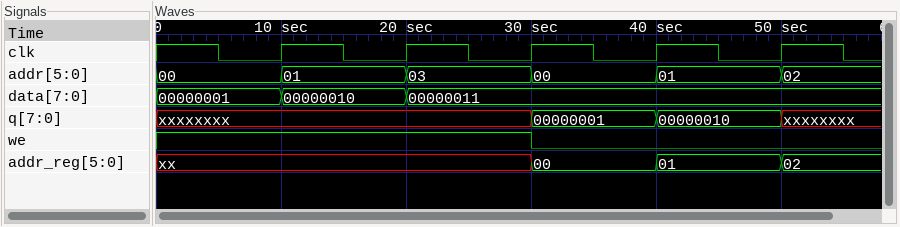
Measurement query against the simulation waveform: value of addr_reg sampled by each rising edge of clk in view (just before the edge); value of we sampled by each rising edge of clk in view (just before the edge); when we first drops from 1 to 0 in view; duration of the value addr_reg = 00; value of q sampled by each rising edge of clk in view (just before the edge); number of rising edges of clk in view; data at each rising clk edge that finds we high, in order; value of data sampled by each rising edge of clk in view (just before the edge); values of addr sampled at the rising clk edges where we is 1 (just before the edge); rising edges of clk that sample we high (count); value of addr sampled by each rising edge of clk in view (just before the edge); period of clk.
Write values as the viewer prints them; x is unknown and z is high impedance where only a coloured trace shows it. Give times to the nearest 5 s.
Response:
xx, xx, xx, 00, 01
1 1 1 0 0
30 s
10 s
xxxxxxxx, xxxxxxxx, xxxxxxxx, 00000001, 00000010
5
00000001, 00000010, 00000011
00000001, 00000010, 00000011, 00000011, 00000011
00, 01, 03
3
00, 01, 03, 00, 01
10 s
